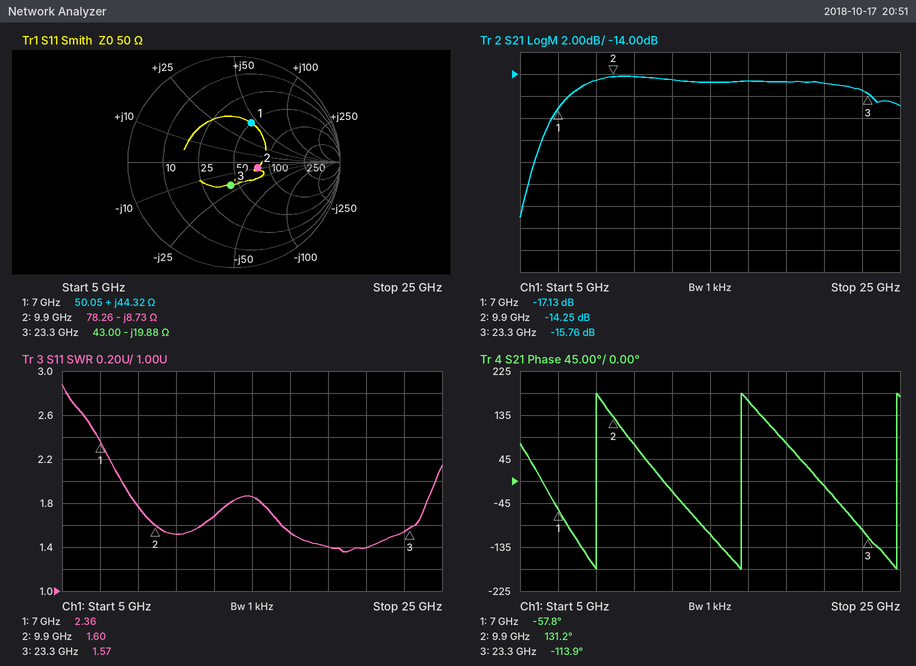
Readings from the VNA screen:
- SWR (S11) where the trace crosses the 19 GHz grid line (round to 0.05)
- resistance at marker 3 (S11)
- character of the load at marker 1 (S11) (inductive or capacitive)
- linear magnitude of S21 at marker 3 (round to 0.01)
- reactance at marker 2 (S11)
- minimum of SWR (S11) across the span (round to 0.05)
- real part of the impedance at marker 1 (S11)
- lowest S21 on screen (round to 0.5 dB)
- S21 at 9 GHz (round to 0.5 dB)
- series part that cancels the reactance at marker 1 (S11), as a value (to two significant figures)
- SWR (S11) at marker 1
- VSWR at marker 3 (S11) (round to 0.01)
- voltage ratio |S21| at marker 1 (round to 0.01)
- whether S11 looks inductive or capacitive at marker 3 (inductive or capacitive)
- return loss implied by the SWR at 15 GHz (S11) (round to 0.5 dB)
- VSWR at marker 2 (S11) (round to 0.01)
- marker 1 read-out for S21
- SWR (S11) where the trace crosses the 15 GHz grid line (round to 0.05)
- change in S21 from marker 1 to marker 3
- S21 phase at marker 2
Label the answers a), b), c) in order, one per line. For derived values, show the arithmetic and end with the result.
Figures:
a) 1.40
b) 43.00 Ω
c) inductive
d) 10^(-15.76/20) ≈ 0.16
e) -8.73 Ω
f) 1.35
g) 50.05 Ω
h) -27.0 dB
i) -14.5 dB
j) C = 1/(2π × 7 GHz × 44.32 Ω) ≈ 513 fF, so 510 fF to two significant figures
k) 2.36
l) 1.57
m) 10^(-17.13/20) ≈ 0.14
n) capacitive
o) −20 log10((1.85 − 1)/(1.85 + 1)) ≈ 10.5 dB
p) 1.60
q) -17.13 dB
r) 1.85
s) -15.76 − (-17.13) = 1.37 dB
t) 131.2°
